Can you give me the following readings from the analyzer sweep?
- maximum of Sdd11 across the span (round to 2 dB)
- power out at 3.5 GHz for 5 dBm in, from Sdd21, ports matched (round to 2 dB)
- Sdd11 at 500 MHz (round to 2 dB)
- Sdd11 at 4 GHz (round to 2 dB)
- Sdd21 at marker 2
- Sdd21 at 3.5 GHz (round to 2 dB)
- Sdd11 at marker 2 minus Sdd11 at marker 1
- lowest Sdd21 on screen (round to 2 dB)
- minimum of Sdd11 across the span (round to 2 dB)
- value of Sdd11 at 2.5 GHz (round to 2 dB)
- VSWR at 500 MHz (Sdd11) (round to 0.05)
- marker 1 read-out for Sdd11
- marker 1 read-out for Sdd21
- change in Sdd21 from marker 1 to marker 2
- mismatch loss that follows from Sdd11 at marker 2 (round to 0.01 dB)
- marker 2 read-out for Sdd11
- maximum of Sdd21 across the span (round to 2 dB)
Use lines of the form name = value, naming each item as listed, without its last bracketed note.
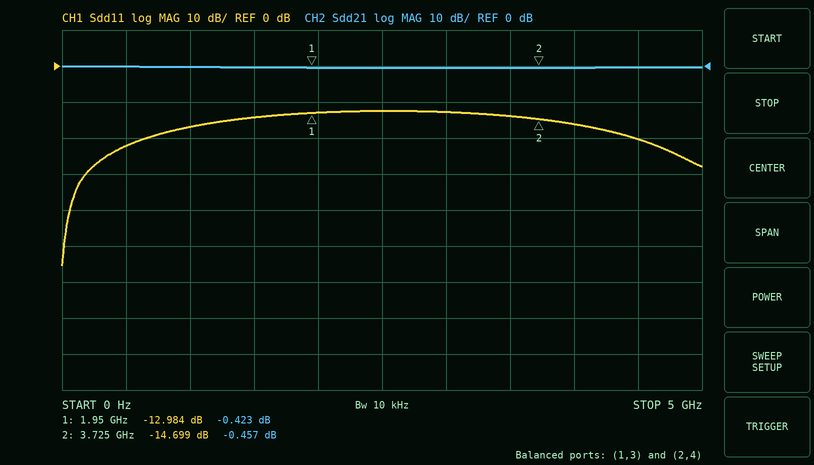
maximum of Sdd11 across the span = -12 dB
power out at 3.5 GHz for 5 dBm in, from Sdd21, ports matched = 4 dBm
Sdd11 at 500 MHz = -22 dB
Sdd11 at 4 GHz = -16 dB
Sdd21 at marker 2 = -0.457 dB
Sdd21 at 3.5 GHz = 0 dB
Sdd11 at marker 2 minus Sdd11 at marker 1 = -1.715 dB
lowest Sdd21 on screen = 0 dB
minimum of Sdd11 across the span = -56 dB
value of Sdd11 at 2.5 GHz = -12 dB
VSWR at 500 MHz (Sdd11) = 1.15
marker 1 read-out for Sdd11 = -12.984 dB
marker 1 read-out for Sdd21 = -0.423 dB
change in Sdd21 from marker 1 to marker 2 = -0.034 dB
mismatch loss that follows from Sdd11 at marker 2 = 0.15 dB
marker 2 read-out for Sdd11 = -14.699 dB
maximum of Sdd21 across the span = 0 dB
